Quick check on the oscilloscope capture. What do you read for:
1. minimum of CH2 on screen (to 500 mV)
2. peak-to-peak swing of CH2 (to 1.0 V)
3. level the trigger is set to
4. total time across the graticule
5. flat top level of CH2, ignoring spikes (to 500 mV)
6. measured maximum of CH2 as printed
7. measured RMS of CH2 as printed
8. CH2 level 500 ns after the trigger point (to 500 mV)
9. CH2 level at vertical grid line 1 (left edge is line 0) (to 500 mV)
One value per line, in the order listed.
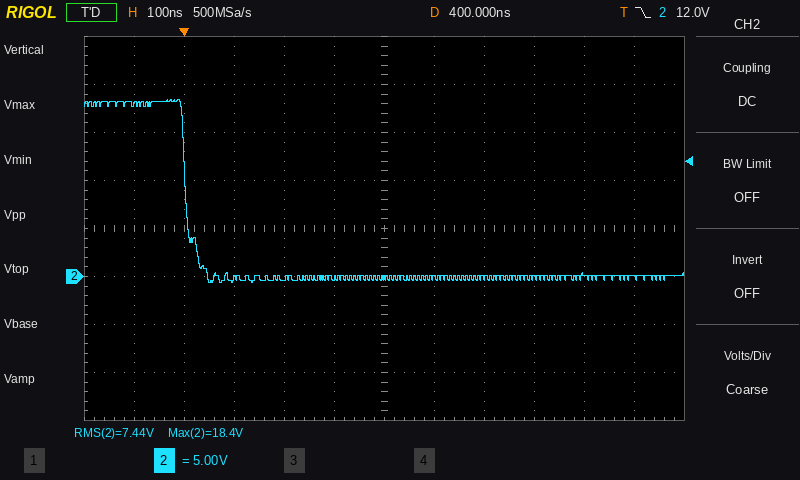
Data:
-500 mV
19.0 V
12.0 V
1.2 µs
18.0 V
18.4 V
7.44 V
0.0 V
18.0 V
